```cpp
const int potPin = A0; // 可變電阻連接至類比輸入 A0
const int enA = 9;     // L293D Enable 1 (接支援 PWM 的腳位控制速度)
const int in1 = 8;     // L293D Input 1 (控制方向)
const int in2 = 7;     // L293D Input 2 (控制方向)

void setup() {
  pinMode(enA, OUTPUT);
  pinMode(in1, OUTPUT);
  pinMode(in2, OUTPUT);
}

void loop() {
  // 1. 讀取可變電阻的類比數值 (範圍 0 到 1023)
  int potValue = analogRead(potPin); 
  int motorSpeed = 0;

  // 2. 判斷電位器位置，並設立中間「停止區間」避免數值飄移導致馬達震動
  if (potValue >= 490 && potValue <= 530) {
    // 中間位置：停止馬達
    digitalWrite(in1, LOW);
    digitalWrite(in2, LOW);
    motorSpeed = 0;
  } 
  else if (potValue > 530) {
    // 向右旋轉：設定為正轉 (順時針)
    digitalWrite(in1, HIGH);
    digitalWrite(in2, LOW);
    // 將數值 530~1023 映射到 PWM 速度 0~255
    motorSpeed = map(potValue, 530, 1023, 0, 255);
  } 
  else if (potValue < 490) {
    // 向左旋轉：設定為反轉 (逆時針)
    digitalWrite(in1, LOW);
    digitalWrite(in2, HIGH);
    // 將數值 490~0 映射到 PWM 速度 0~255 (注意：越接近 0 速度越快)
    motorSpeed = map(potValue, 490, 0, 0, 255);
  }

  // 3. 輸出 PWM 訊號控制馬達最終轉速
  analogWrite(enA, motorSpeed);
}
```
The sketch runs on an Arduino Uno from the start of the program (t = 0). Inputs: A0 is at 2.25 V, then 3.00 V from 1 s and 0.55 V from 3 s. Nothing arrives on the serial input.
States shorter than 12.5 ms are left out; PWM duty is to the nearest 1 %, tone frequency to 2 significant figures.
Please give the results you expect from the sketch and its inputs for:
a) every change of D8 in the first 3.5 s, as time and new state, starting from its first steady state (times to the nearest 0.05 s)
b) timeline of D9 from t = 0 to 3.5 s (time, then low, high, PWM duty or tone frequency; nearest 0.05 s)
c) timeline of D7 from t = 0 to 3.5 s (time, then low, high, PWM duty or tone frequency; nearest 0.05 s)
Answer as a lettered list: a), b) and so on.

a) 0 s low; 1 s high; 3 s low
b) 0 s PWM 6 %; 1 s PWM 17 %; 3 s PWM 77 %
c) 0 s high; 1 s low; 3 s high
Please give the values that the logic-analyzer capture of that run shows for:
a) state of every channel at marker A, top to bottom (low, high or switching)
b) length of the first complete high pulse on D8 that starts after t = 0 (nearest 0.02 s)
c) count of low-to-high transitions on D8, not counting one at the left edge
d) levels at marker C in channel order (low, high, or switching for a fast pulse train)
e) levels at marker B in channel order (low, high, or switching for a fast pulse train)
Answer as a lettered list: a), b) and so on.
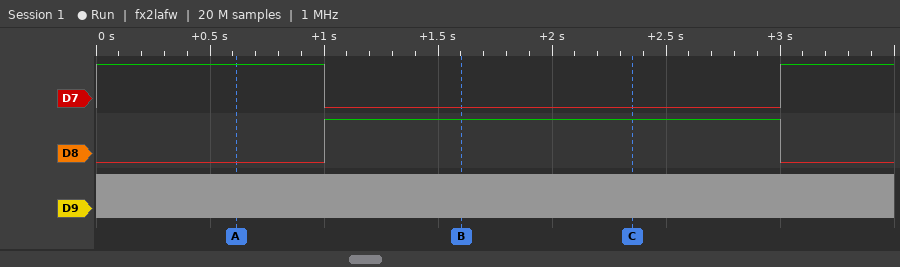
a) D7 high, D8 low, D9 switching
b) 2.00 s
c) 1
d) D7 low, D8 high, D9 switching
e) D7 low, D8 high, D9 switching
